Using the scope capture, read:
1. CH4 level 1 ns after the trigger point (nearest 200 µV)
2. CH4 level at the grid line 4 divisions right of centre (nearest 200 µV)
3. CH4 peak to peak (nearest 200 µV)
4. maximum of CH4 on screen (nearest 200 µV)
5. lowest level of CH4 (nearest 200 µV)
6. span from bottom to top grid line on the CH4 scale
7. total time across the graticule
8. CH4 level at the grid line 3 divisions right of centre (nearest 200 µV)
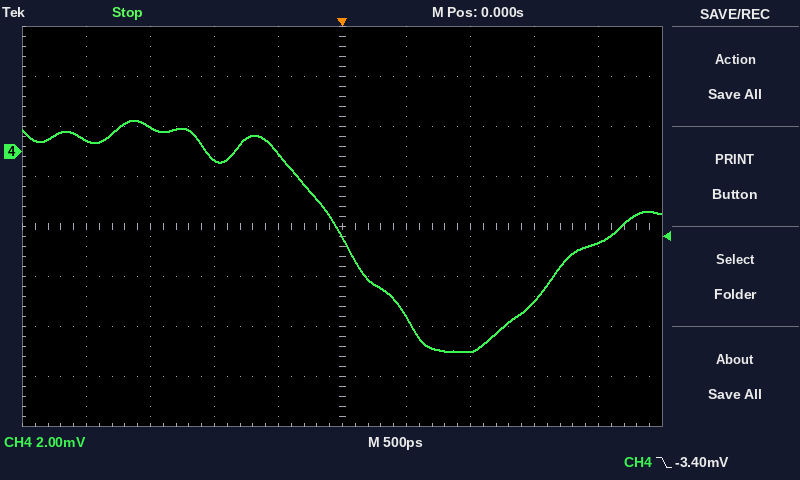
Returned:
-8.0 mV
-3.6 mV
9.2 mV
1.2 mV
-8.0 mV
16 mV
5 ns
-6.0 mV
